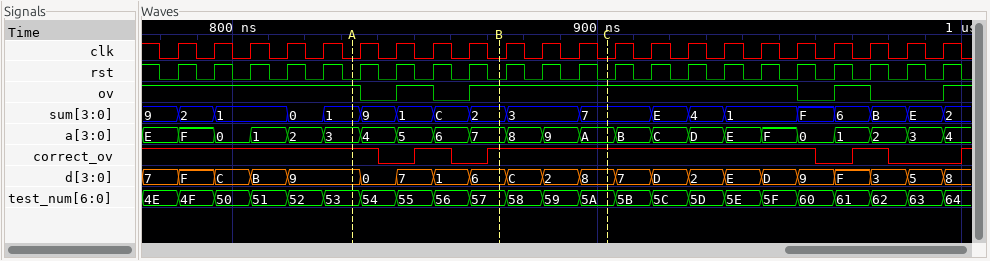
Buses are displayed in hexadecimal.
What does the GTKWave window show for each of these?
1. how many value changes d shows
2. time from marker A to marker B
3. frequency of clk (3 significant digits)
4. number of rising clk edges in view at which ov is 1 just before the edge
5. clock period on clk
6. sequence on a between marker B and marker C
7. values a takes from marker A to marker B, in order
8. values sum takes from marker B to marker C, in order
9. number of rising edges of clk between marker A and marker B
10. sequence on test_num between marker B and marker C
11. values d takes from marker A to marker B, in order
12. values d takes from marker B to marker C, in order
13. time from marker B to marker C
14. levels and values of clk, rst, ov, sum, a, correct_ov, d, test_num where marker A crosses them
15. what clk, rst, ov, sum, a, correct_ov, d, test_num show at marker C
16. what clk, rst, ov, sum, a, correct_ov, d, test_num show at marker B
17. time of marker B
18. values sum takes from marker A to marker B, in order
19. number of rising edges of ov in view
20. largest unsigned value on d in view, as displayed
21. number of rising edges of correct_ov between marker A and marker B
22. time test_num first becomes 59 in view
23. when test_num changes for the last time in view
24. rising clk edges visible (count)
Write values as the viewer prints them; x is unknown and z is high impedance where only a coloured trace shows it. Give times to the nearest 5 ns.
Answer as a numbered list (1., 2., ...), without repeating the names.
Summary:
1. 21
2. 40 ns
3. 100 MHz
4. 17
5. 10 ns
6. 7, 8, 9, A
7. 3, 4, 5, 6, 7
8. 2, 3, 7
9. 4
10. 57, 58, 59, 5A
11. 9, 0, 7, 1, 6
12. 6, C, 2, 8
13. 30 ns
14. clk=0, rst=0, ov=1, sum=1, a=3, correct_ov=1, d=9, test_num=53
15. clk=0, rst=0, ov=1, sum=7, a=A, correct_ov=1, d=8, test_num=5A
16. clk=0, rst=0, ov=1, sum=2, a=7, correct_ov=1, d=6, test_num=57
17. 875 ns
18. 1, 9, 1, C, 2
19. 4
20. F
21. 2
22. 885 ns
23. 995 ns
24. 22
